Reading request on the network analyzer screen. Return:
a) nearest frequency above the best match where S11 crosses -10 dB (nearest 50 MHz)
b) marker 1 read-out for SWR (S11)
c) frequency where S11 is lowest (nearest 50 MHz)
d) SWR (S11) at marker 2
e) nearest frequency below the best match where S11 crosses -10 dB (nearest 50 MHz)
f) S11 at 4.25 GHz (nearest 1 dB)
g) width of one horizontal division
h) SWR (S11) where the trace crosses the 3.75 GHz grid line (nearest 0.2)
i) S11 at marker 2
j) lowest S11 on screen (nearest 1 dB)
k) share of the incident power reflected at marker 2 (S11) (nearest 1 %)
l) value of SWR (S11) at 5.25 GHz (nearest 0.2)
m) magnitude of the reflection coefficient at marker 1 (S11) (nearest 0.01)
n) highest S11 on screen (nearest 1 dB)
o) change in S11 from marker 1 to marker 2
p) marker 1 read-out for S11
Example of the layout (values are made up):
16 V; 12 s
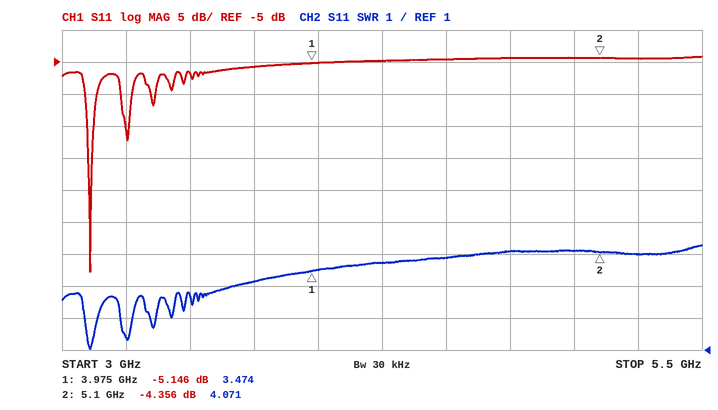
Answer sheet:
3.15 GHz; 3.474; 3.10 GHz; 4.071; 3.10 GHz; -5 dB; 250 MHz; 3.2; -4.356 dB; -38 dB; 37 %; 4.0; 0.55; -4 dB; 0.790 dB; -5.146 dB
